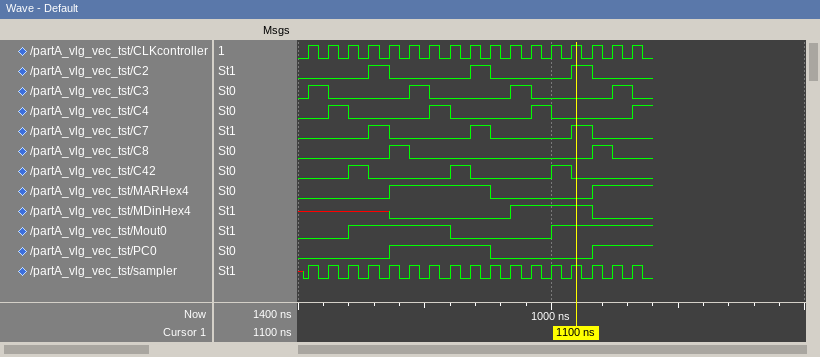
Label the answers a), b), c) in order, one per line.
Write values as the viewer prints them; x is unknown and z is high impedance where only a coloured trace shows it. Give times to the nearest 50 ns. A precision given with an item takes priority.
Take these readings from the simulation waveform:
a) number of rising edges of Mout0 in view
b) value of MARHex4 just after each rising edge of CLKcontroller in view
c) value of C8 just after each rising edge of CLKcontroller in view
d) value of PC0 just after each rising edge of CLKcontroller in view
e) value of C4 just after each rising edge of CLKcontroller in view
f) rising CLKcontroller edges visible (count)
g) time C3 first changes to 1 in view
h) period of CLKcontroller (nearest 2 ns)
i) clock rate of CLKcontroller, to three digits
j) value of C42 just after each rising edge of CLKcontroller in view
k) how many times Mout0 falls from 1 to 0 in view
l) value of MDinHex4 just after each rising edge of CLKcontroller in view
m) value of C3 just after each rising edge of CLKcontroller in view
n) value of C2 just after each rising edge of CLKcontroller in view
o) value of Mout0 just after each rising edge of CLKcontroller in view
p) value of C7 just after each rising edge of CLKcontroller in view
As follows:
a) 2
b) 0 0 0 0 1 1 1 1 1 0 0 0 0 0 1 1 1
c) 0 0 0 0 1 0 0 0 0 0 0 0 0 0 1 0 0
d) 0 0 0 0 1 1 1 1 1 0 0 0 0 0 1 1 1
e) 0 1 0 0 0 0 1 0 0 0 0 1 0 0 0 0 1
f) 17
g) 50 ns
h) 80 ns
i) 12.5 MHz
j) 0 0 1 0 0 0 0 1 0 0 0 0 1 0 0 0 0
k) 1
l) x x x x 0 0 0 0 0 0 1 1 1 1 0 0 0
m) 1 0 0 0 0 1 0 0 0 0 1 0 0 0 0 1 0
n) 0 0 0 1 0 0 0 0 1 0 0 0 0 1 0 0 0
o) 0 0 1 1 1 1 1 0 0 0 0 0 1 1 1 1 1
p) 0 0 0 1 0 0 0 0 1 0 0 0 0 1 0 0 0
